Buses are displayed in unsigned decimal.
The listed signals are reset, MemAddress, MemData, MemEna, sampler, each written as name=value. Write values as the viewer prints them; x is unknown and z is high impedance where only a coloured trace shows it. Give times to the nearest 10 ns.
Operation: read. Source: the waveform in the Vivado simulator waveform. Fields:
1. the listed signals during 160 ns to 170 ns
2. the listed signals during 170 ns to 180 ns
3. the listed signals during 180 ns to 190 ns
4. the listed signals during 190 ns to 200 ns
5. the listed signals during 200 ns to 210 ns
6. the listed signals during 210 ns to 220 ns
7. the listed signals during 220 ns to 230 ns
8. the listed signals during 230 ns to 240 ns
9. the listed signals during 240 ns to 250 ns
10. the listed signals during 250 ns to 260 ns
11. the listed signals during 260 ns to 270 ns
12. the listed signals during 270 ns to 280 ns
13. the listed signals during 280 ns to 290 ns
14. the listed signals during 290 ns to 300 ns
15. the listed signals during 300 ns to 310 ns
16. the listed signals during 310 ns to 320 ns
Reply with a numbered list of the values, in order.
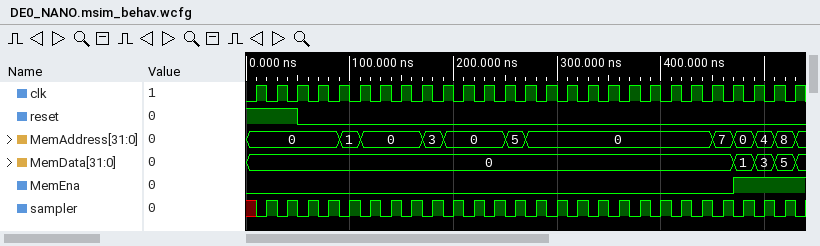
1. reset=0, MemAddress=0, MemData=0, MemEna=0, sampler=1
2. reset=0, MemAddress=3, MemData=0, MemEna=0, sampler=0
3. reset=0, MemAddress=3, MemData=0, MemEna=0, sampler=1
4. reset=0, MemAddress=0, MemData=0, MemEna=0, sampler=0
5. reset=0, MemAddress=0, MemData=0, MemEna=0, sampler=1
6. reset=0, MemAddress=0, MemData=0, MemEna=0, sampler=0
7. reset=0, MemAddress=0, MemData=0, MemEna=0, sampler=1
8. reset=0, MemAddress=0, MemData=0, MemEna=0, sampler=0
9. reset=0, MemAddress=0, MemData=0, MemEna=0, sampler=1
10. reset=0, MemAddress=5, MemData=0, MemEna=0, sampler=0
11. reset=0, MemAddress=5, MemData=0, MemEna=0, sampler=1
12. reset=0, MemAddress=0, MemData=0, MemEna=0, sampler=0
13. reset=0, MemAddress=0, MemData=0, MemEna=0, sampler=1
14. reset=0, MemAddress=0, MemData=0, MemEna=0, sampler=0
15. reset=0, MemAddress=0, MemData=0, MemEna=0, sampler=1
16. reset=0, MemAddress=0, MemData=0, MemEna=0, sampler=0
